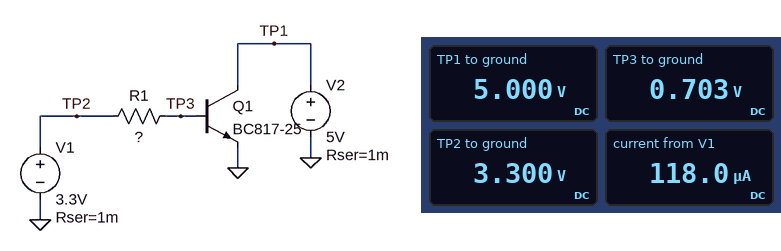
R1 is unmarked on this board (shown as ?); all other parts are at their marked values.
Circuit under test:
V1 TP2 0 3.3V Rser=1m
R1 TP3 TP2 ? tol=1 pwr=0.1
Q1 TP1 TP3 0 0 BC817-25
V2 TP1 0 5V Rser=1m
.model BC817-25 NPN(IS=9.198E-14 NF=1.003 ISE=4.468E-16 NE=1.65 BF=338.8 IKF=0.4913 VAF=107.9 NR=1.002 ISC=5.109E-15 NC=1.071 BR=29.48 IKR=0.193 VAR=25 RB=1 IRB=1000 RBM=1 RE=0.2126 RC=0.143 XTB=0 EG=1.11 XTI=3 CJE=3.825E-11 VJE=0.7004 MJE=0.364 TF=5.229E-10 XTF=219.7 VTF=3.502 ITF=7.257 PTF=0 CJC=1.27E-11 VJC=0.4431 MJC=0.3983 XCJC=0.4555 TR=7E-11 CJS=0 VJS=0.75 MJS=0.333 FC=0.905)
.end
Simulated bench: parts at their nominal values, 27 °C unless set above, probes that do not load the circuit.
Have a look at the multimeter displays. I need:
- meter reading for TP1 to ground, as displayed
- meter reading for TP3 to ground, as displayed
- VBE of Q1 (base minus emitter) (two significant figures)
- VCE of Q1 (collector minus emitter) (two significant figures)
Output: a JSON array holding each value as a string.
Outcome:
["5.000 V", "0.703 V", "700 mV", "5.0 V"]
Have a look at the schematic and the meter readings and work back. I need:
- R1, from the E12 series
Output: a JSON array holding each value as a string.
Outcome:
["22 kΩ"]
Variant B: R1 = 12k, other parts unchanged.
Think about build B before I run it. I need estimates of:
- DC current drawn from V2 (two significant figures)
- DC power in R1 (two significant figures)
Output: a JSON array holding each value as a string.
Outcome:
["65 mA", "550 µW"]
